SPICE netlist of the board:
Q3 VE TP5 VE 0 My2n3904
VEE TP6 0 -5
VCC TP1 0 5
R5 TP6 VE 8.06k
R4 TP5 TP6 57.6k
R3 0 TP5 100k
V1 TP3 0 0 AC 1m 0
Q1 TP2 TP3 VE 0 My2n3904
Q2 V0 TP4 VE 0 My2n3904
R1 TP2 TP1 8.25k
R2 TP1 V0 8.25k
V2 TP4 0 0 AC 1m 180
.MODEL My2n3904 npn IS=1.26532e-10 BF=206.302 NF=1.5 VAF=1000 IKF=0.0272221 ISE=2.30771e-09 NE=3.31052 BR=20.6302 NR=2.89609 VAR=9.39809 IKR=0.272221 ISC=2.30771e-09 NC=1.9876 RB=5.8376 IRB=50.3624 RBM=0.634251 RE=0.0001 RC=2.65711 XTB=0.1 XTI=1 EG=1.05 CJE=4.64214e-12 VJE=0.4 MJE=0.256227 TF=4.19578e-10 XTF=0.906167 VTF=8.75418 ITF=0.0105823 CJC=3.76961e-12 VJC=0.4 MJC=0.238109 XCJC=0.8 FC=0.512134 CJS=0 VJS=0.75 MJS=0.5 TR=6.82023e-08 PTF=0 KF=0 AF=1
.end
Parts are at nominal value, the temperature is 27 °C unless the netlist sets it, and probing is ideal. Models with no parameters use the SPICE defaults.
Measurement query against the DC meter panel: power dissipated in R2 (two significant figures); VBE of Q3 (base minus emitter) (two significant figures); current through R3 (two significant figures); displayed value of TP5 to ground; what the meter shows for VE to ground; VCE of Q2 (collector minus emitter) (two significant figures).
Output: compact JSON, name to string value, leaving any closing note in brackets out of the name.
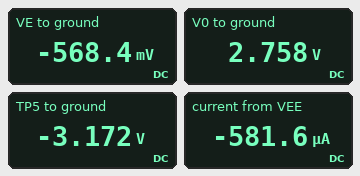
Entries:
{"power dissipated in R2": "610 µW", "VBE of Q3 (base minus emitter)": "-2.6 V", "current through R3": "32 µA", "displayed value of TP5 to ground": "-3.172 V", "what the meter shows for VE to ground": "-568.4 mV", "VCE of Q2 (collector minus emitter)": "3.3 V"}
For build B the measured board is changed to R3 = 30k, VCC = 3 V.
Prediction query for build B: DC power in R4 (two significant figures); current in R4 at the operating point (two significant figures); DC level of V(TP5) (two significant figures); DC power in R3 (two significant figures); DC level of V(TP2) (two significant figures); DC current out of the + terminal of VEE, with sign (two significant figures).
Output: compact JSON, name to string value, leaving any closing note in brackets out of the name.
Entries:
{"DC power in R4": "190 µW", "current in R4 at the operating point": "57 µA", "DC level of V(TP5)": "-1.7 V", "DC power in R3": "98 µW", "DC level of V(TP2)": "760 mV", "DC current out of the + terminal of VEE, with sign": "-610 µA"}
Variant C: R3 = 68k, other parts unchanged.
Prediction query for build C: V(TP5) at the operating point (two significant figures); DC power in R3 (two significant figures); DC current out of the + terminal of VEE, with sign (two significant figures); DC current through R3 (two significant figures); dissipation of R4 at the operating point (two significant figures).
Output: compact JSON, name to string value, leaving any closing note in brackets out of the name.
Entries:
{"V(TP5) at the operating point": "-2.7 V", "DC power in R3": "110 µW", "DC current out of the + terminal of VEE, with sign": "-590 µA", "DC current through R3": "40 µA", "dissipation of R4 at the operating point": "91 µW"}
